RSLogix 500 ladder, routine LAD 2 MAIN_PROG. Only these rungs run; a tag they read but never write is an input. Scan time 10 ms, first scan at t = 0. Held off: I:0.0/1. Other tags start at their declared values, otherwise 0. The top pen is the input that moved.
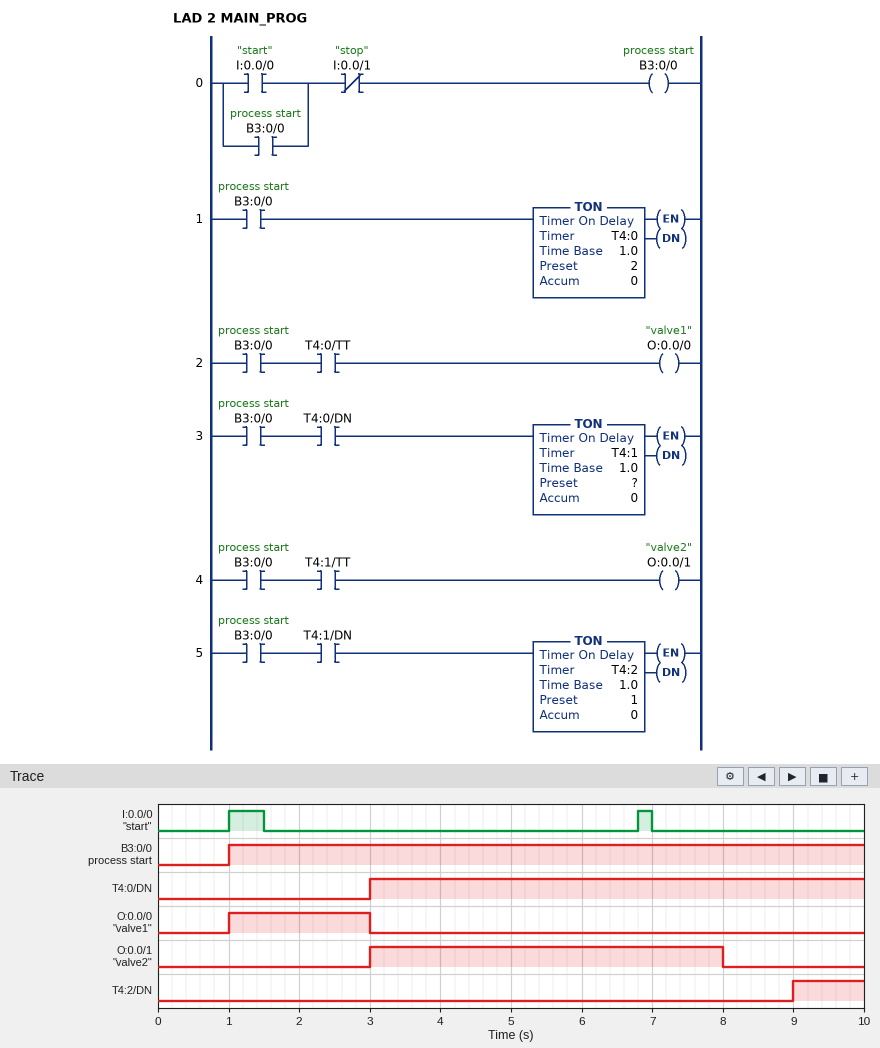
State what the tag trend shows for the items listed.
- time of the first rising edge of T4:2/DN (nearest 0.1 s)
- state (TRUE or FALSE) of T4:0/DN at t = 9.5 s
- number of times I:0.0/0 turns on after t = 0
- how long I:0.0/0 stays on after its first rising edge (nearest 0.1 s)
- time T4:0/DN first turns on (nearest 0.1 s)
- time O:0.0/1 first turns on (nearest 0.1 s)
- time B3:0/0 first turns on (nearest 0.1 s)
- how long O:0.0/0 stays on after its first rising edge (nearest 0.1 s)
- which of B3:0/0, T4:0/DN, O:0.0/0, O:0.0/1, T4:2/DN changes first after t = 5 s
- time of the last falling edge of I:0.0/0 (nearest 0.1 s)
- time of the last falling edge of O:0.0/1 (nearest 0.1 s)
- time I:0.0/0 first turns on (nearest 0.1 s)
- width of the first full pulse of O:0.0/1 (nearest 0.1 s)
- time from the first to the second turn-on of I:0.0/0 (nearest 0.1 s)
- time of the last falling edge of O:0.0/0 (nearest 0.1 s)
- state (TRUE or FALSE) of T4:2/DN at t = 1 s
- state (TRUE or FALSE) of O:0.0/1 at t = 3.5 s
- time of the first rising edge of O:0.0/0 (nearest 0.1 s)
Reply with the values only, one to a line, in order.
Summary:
9.0 s
TRUE
2
0.5 s
3.0 s
3.0 s
1.0 s
2.0 s
O:0.0/1
7.0 s
8.0 s
1.0 s
5.0 s
5.8 s
3.0 s
FALSE
TRUE
1.0 s
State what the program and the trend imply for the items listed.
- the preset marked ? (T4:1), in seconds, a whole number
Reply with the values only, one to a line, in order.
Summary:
5 s
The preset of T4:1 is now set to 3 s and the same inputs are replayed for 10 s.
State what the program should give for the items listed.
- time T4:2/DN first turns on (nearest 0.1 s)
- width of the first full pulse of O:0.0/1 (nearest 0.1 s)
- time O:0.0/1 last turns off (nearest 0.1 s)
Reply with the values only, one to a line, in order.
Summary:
7.0 s
3.0 s
6.0 s
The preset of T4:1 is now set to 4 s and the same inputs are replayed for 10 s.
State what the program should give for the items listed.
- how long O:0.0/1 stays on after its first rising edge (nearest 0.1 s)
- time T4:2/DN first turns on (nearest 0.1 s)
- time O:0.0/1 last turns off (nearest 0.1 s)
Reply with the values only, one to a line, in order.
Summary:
4.0 s
8.0 s
7.0 s
